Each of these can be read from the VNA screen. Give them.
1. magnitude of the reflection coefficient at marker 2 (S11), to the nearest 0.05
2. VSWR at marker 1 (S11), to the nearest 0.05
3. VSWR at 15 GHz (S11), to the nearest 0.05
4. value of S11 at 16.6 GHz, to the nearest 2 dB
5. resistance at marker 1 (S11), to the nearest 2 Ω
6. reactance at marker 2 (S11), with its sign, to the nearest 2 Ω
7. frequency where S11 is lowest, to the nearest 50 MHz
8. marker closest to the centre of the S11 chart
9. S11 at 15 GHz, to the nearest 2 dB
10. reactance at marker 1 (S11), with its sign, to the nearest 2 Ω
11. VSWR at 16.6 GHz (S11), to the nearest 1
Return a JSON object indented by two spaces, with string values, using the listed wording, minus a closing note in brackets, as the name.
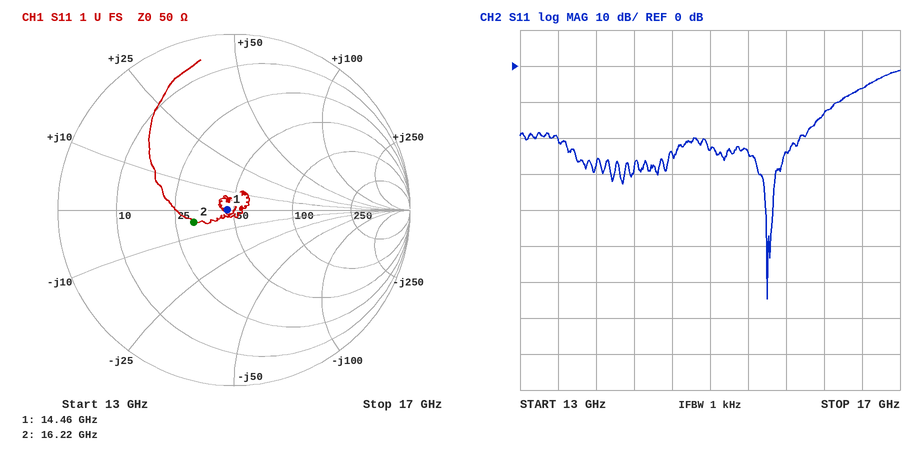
{
  "magnitude of the reflection coefficient at marker 2 (S11), to the nearest 0.05": "0.25",
  "VSWR at marker 1 (S11), to the nearest 0.05": "1.10",
  "VSWR at 15 GHz (S11), to the nearest 0.05": "1.15",
  "value of S11 at 16.6 GHz, to the nearest 2 dB": "-6 dB",
  "resistance at marker 1 (S11), to the nearest 2 Ω": "46 Ω",
  "reactance at marker 2 (S11), with its sign, to the nearest 2 Ω": "-4 Ω",
  "frequency where S11 is lowest, to the nearest 50 MHz": "15.60 GHz",
  "marker closest to the centre of the S11 chart": "marker 1",
  "S11 at 15 GHz, to the nearest 2 dB": "-24 dB",
  "reactance at marker 1 (S11), with its sign, to the nearest 2 Ω": "0 Ω",
  "VSWR at 16.6 GHz (S11), to the nearest 1": "3"
}
